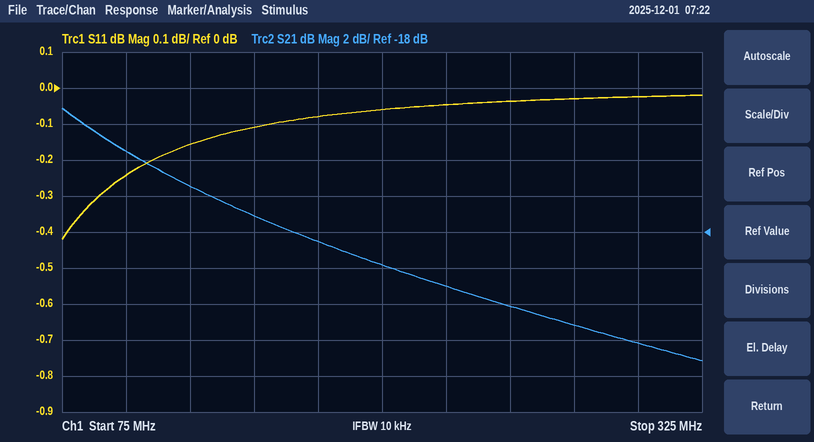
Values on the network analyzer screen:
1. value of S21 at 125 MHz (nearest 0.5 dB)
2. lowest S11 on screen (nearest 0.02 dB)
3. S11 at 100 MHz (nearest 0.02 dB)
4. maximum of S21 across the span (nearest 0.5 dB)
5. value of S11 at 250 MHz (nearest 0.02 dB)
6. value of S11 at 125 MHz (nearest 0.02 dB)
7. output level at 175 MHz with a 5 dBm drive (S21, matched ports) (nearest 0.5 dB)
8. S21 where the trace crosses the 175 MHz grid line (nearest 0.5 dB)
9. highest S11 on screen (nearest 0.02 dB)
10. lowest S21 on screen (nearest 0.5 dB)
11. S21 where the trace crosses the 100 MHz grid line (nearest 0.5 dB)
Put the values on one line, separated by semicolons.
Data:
-15.5 dB; -0.42 dB; -0.24 dB; -11.0 dB; -0.04 dB; -0.16 dB; -13.5 dBm; -18.5 dB; -0.02 dB; -25.0 dB; -13.5 dB
